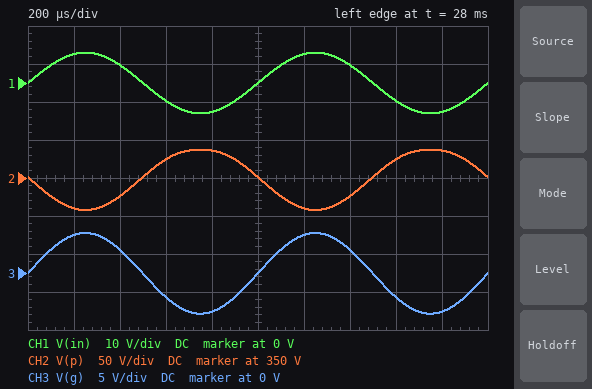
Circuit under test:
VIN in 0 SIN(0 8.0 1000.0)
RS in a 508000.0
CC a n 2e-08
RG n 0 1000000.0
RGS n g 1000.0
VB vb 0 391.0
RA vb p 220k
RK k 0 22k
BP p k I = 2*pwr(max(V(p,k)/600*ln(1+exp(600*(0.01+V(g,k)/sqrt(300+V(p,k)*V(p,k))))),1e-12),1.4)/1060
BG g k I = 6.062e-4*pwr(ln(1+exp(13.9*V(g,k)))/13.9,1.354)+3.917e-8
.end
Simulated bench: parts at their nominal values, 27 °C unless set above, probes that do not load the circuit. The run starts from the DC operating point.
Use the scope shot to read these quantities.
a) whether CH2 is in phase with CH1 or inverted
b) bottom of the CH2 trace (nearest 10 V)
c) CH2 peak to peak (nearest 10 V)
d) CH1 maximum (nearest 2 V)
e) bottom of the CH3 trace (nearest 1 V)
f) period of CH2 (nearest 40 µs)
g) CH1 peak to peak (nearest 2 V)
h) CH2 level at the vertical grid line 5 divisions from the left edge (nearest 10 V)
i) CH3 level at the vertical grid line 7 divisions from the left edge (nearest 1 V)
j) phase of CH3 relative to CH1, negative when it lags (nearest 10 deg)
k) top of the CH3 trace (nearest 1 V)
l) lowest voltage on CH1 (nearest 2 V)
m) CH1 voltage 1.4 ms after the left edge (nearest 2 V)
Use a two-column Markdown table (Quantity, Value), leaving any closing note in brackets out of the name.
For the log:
| Quantity | Value |
|---|---|
| whether CH2 is in phase with CH1 or inverted | inverted |
| bottom of the CH2 trace | 310 V |
| CH2 peak to peak | 80 V |
| CH1 maximum | 8 V |
| bottom of the CH3 trace | -5 V |
| period of CH2 | 1.00 ms |
| CH1 peak to peak | 16 V |
| CH2 level at the vertical grid line 5 divisions from the left edge | 350 V |
| CH3 level at the vertical grid line 7 divisions from the left edge | 3 V |
| phase of CH3 relative to CH1, negative when it lags | 0 deg |
| top of the CH3 trace | 5 V |
| lowest voltage on CH1 | -8 V |
| CH1 voltage 1.4 ms after the left edge | 4 V |
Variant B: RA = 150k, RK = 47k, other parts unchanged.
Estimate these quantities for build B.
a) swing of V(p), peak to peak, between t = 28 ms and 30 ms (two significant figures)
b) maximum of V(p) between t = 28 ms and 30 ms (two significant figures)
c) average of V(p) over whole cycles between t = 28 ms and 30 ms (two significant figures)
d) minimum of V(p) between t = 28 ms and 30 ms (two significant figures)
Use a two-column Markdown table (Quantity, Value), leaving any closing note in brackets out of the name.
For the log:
| Quantity | Value |
|---|---|
| swing of V(p), peak to peak, between t = 28 ms and 30 ms | 28 V |
| maximum of V(p) between t = 28 ms and 30 ms | 390 V |
| average of V(p) over whole cycles between t = 28 ms and 30 ms | 380 V |
| minimum of V(p) between t = 28 ms and 30 ms | 360 V |
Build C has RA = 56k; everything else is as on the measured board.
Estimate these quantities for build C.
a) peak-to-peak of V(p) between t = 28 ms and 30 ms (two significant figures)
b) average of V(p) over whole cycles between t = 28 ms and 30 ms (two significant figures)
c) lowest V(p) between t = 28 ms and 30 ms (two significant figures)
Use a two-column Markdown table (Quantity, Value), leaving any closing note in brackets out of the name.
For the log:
| Quantity | Value |
|---|---|
| peak-to-peak of V(p) between t = 28 ms and 30 ms | 22 V |
| average of V(p) over whole cycles between t = 28 ms and 30 ms | 380 V |
| lowest V(p) between t = 28 ms and 30 ms | 370 V |
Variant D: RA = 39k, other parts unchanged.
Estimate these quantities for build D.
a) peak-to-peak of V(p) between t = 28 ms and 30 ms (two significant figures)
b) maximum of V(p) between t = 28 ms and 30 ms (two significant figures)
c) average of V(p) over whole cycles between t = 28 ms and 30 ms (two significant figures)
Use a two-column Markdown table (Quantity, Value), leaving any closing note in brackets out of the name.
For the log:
| Quantity | Value |
|---|---|
| peak-to-peak of V(p) between t = 28 ms and 30 ms | 15 V |
| maximum of V(p) between t = 28 ms and 30 ms | 390 V |
| average of V(p) over whole cycles between t = 28 ms and 30 ms | 380 V |
